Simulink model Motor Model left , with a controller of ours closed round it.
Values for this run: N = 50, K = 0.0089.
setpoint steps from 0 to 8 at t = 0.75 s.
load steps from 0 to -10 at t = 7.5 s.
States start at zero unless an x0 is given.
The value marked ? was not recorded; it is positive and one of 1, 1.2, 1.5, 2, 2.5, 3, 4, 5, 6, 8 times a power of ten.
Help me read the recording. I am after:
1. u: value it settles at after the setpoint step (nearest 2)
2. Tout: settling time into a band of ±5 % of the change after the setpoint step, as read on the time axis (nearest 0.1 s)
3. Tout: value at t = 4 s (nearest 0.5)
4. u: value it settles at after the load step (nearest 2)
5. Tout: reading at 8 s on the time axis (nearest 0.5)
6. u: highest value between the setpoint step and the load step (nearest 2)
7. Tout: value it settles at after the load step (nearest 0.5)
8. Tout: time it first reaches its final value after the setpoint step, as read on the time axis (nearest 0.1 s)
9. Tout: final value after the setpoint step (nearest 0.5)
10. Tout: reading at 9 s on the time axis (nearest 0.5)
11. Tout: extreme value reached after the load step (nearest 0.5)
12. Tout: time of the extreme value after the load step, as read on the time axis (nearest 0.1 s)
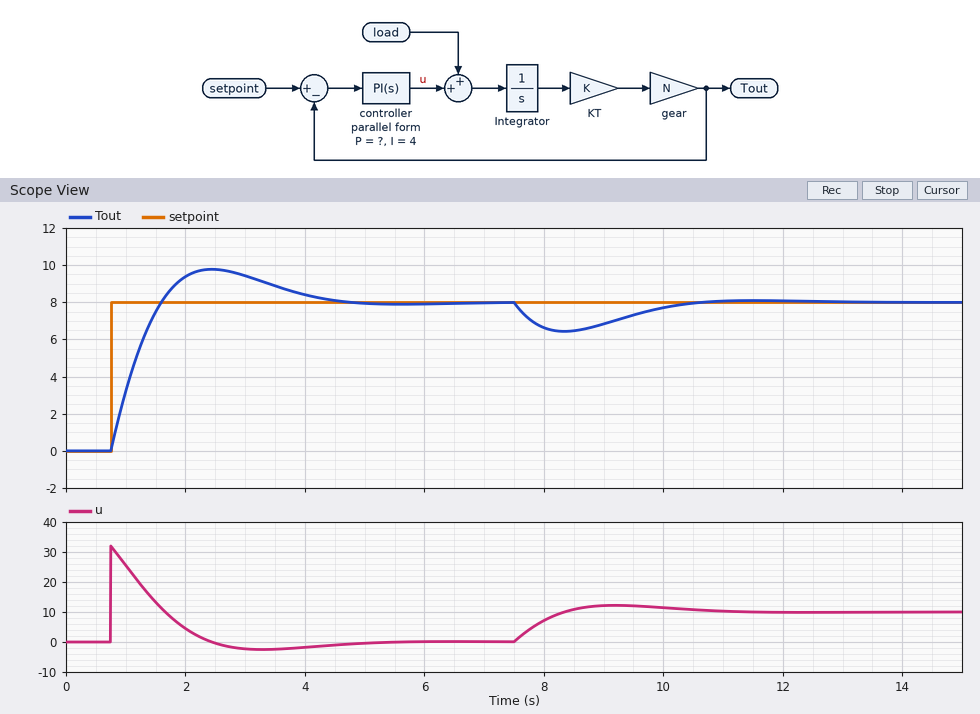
0
4.0 s
8.5
10
6.5
32
8.0
1.6 s
8.0
7.0
6.5
8.3 s
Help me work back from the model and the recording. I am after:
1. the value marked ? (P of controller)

4
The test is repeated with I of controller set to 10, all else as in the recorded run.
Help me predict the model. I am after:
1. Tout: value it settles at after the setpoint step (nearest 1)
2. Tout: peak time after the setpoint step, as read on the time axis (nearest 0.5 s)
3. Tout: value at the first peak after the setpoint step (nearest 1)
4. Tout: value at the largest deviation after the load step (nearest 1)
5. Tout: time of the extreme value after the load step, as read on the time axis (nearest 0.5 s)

8
2.0 s
11
7
8.0 s
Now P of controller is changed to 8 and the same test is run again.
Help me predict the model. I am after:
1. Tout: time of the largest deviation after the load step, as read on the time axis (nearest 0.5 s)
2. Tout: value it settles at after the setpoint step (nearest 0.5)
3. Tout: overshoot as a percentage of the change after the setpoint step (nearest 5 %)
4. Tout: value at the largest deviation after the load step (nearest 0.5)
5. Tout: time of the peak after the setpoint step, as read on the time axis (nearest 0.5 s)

8.0 s
8.0
10 %
7.0
2.0 s
